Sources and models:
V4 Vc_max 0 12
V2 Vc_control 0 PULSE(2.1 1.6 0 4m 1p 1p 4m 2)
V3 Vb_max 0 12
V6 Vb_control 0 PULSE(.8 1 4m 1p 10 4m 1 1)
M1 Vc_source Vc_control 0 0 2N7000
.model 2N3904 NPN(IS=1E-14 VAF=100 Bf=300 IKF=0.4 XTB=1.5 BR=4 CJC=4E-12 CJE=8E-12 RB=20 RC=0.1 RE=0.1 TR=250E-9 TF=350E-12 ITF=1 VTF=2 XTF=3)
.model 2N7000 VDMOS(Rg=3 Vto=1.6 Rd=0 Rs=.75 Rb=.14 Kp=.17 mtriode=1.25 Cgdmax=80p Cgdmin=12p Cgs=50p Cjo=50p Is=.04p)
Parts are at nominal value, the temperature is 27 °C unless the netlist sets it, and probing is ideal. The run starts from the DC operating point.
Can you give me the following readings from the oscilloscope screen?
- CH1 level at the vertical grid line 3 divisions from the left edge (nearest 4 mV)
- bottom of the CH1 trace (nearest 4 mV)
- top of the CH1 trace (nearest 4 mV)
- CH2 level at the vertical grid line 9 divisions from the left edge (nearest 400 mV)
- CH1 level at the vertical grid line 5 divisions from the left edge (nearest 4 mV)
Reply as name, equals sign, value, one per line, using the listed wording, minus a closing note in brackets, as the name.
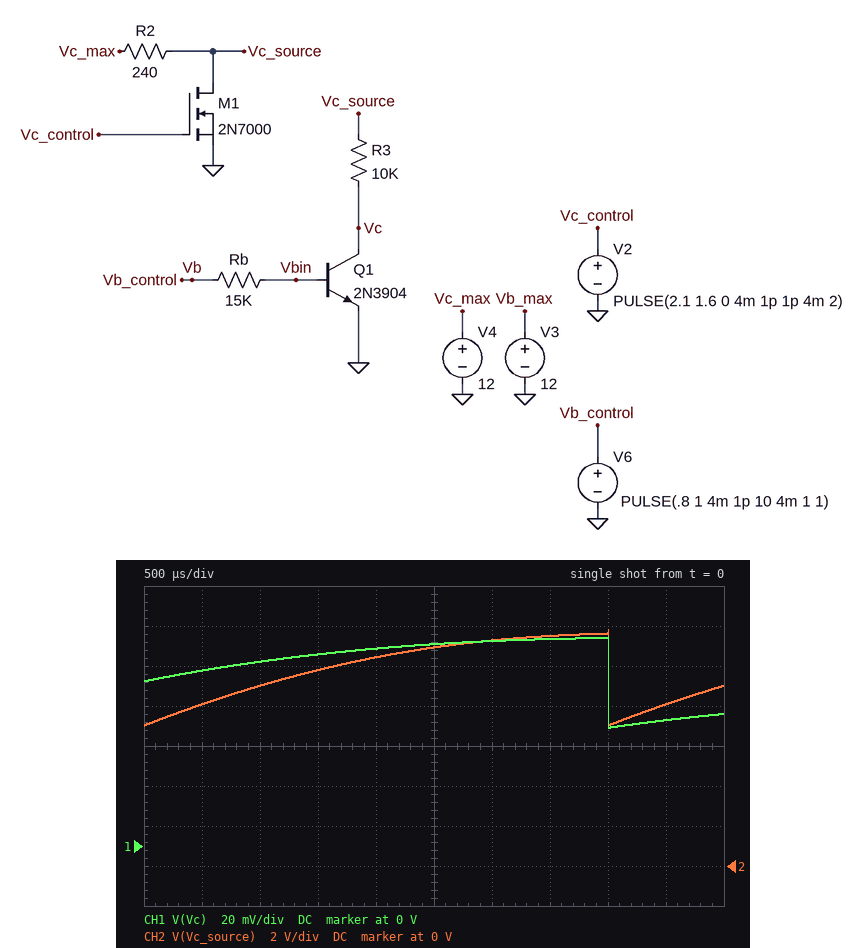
CH1 level at the vertical grid line 3 divisions from the left edge = 96 mV
bottom of the CH1 trace = 60 mV
top of the CH1 trace = 104 mV
CH2 level at the vertical grid line 9 divisions from the left edge = 8.0 V
CH1 level at the vertical grid line 5 divisions from the left edge = 100 mV
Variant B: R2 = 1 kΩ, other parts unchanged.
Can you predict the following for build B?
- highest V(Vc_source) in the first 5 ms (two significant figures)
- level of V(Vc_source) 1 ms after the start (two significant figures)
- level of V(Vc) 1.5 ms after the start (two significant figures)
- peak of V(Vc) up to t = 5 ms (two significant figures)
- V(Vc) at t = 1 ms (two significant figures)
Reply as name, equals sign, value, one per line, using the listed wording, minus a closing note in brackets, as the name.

highest V(Vc_source) in the first 5 ms = 11 V
level of V(Vc_source) 1 ms after the start = 400 mV
level of V(Vc) 1.5 ms after the start = 59 mV
peak of V(Vc) up to t = 5 ms = 100 mV
V(Vc) at t = 1 ms = 18 mV
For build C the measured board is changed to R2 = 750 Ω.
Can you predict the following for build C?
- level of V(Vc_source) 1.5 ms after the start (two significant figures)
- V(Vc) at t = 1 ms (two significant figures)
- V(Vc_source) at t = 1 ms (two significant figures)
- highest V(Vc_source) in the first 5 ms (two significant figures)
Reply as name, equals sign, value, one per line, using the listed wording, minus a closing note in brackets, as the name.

level of V(Vc_source) 1.5 ms after the start = 5.4 V
V(Vc) at t = 1 ms = 56 mV
V(Vc_source) at t = 1 ms = 3.1 V
highest V(Vc_source) in the first 5 ms = 11 V
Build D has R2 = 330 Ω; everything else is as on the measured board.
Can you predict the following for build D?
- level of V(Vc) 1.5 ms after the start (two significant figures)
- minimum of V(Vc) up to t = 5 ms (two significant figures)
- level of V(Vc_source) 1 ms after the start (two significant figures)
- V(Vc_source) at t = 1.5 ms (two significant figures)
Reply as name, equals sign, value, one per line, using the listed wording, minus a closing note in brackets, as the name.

level of V(Vc) 1.5 ms after the start = 92 mV
minimum of V(Vc) up to t = 5 ms = 51 mV
level of V(Vc_source) 1 ms after the start = 7.9 V
V(Vc_source) at t = 1.5 ms = 9.0 V
